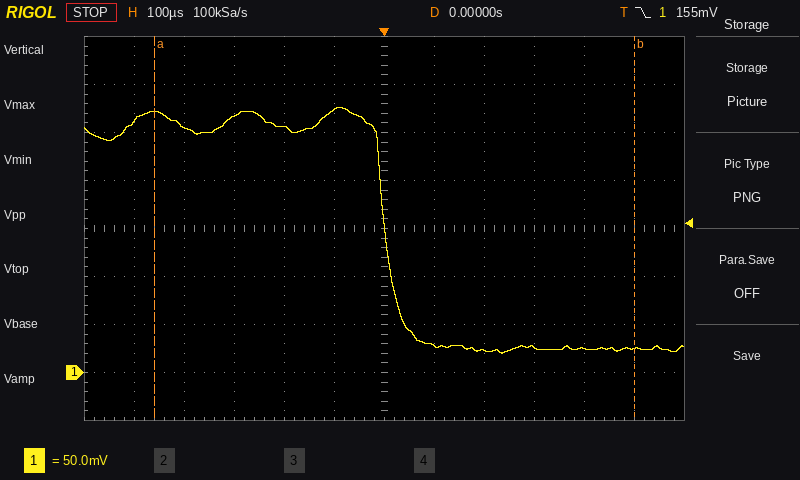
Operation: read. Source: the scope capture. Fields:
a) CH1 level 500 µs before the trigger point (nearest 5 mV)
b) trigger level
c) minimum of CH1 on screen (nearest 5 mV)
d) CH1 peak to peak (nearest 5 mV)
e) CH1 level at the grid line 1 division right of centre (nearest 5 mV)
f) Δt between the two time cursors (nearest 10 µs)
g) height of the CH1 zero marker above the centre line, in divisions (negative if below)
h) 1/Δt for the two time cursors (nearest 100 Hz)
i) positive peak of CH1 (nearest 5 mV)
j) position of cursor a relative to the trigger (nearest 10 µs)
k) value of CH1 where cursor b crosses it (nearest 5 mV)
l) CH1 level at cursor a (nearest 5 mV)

260 mV
155 mV
20 mV
255 mV
30 mV
960 µs
-3.0 div
1.0 kHz
275 mV
-460 µs
25 mV
270 mV
